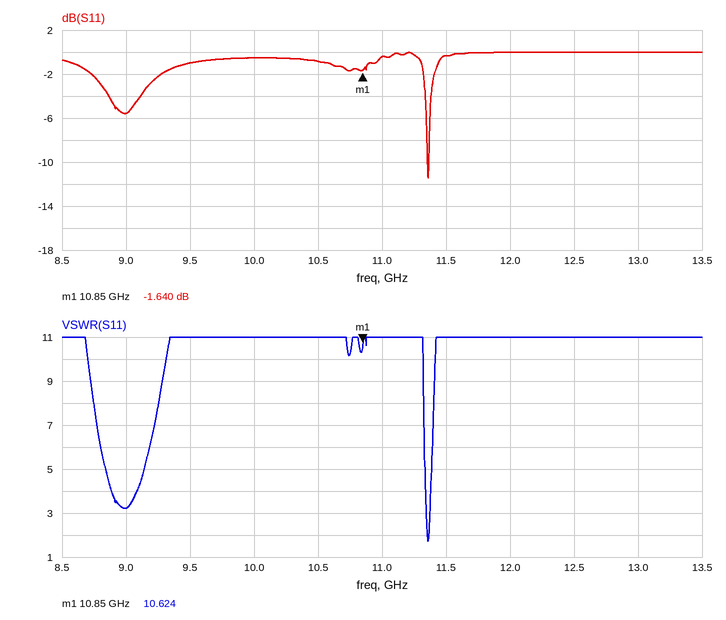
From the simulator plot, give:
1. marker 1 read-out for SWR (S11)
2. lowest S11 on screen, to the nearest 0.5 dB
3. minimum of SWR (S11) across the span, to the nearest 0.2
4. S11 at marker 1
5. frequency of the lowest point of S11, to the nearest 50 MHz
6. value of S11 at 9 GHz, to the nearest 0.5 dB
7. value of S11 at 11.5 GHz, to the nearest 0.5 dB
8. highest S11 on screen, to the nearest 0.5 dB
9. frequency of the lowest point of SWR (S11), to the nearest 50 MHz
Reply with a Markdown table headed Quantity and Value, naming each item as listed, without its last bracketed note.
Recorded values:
| Quantity | Value |
|---|---|
| marker 1 read-out for SWR | 10.624 |
| lowest S11 on screen, to the nearest 0.5 dB | -11.5 dB |
| minimum of SWR (S11) across the span, to the nearest 0.2 | 1.8 |
| S11 at marker 1 | -1.640 dB |
| frequency of the lowest point of S11, to the nearest 50 MHz | 11.35 GHz |
| value of S11 at 9 GHz, to the nearest 0.5 dB | -5.5 dB |
| value of S11 at 11.5 GHz, to the nearest 0.5 dB | -0.5 dB |
| highest S11 on screen, to the nearest 0.5 dB | 0.0 dB |
| frequency of the lowest point of SWR (S11), to the nearest 50 MHz | 11.35 GHz |
